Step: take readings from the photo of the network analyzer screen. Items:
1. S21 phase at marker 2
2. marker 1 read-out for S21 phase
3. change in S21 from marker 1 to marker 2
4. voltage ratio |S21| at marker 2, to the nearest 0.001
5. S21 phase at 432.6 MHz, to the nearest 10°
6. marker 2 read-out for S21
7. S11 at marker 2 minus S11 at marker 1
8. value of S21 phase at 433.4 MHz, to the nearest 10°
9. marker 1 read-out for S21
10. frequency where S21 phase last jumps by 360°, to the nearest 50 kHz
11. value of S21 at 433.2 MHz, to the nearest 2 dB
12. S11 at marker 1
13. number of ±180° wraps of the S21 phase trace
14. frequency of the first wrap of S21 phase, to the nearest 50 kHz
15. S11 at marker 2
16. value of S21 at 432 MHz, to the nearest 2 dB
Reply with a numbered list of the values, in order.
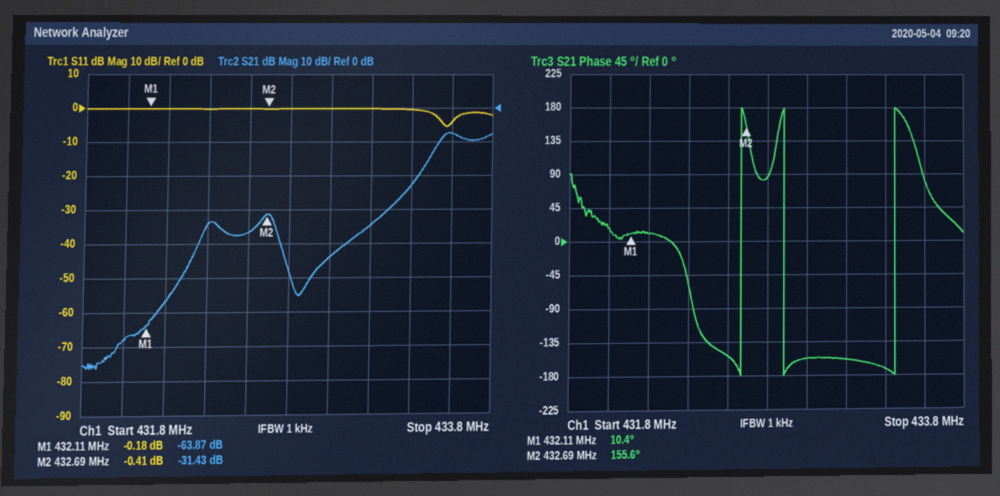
1. 155.6°
2. 10.4°
3. 32.44 dB
4. 0.027
5. -150°
6. -31.43 dB
7. -0.23 dB
8. -170°
9. -63.87 dB
10. 433.45 MHz
11. -34 dB
12. -0.18 dB
13. 3
14. 432.65 MHz
15. -0.41 dB
16. -68 dB
